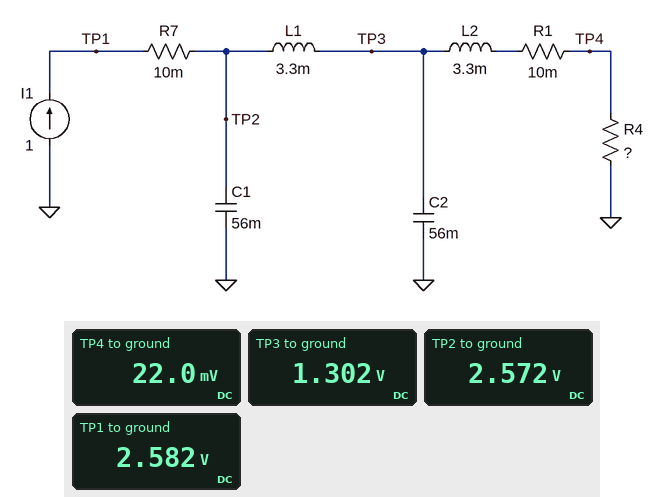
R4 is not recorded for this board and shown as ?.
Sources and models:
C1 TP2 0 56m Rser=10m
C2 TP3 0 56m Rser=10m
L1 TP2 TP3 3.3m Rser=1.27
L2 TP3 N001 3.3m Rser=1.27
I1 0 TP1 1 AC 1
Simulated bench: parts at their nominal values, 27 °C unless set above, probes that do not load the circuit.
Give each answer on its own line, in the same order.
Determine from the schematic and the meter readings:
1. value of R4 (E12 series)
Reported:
0.022 Ω
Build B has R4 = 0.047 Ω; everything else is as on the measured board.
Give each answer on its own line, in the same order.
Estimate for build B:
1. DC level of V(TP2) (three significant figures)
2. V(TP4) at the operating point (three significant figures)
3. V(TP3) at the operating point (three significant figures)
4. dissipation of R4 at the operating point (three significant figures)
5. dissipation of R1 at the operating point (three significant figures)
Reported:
2.60 V
47.0 mV
1.33 V
47.0 mW
10.0 mW
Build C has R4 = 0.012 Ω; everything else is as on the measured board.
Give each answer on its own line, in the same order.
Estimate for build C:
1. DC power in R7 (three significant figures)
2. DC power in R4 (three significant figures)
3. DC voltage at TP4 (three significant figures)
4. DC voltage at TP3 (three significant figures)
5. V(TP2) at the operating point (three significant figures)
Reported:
10.0 mW
12.0 mW
12.0 mV
1.29 V
2.56 V
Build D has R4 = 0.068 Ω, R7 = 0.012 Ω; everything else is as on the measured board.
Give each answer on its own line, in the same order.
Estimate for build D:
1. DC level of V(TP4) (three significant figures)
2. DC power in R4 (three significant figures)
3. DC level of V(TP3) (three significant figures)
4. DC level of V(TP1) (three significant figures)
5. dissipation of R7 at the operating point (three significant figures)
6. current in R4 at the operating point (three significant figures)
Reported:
68.0 mV
68.0 mW
1.35 V
2.63 V
12.0 mW
1.00 A
